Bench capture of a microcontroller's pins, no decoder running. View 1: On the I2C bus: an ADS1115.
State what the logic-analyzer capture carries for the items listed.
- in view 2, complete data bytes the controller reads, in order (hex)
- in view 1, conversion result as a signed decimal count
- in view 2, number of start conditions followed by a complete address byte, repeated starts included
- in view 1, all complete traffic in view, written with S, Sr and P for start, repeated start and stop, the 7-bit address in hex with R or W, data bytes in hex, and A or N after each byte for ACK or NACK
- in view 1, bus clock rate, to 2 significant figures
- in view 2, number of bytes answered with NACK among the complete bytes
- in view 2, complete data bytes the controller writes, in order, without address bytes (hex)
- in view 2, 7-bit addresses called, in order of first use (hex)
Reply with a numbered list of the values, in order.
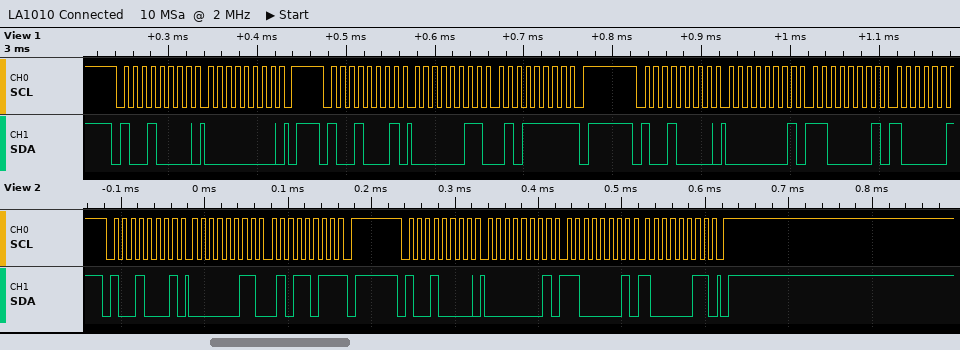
1. 03 5B
2. 863
3. 2
4. S 48W A 00 A P S 48R A 03 A 5F N P S 48W A 01 A C1 A
5. 100 kHz
6. 1
7. 01 C1 83
8. 0x48
